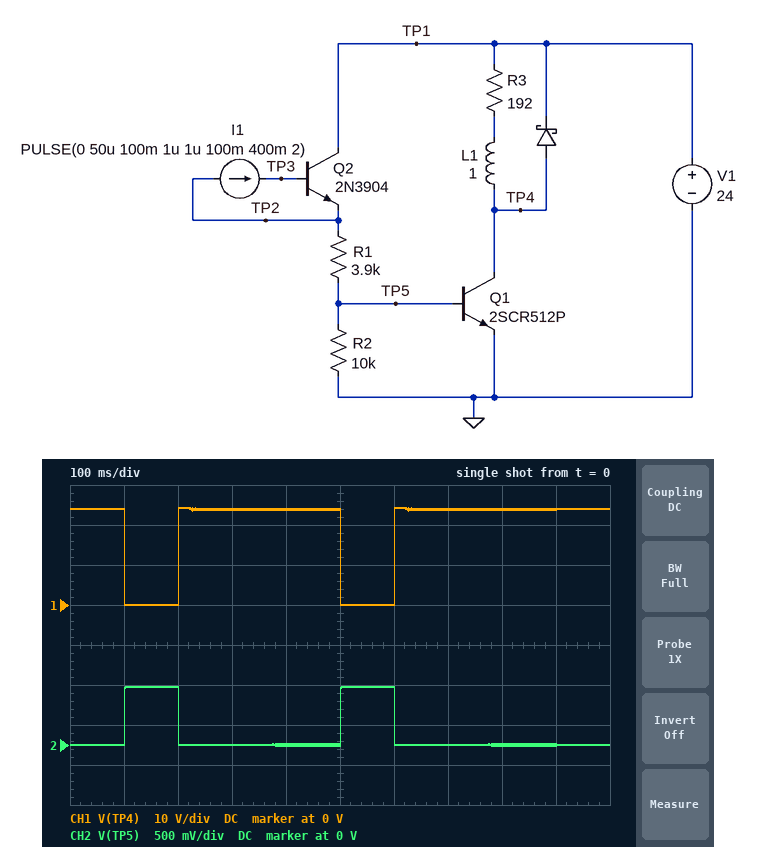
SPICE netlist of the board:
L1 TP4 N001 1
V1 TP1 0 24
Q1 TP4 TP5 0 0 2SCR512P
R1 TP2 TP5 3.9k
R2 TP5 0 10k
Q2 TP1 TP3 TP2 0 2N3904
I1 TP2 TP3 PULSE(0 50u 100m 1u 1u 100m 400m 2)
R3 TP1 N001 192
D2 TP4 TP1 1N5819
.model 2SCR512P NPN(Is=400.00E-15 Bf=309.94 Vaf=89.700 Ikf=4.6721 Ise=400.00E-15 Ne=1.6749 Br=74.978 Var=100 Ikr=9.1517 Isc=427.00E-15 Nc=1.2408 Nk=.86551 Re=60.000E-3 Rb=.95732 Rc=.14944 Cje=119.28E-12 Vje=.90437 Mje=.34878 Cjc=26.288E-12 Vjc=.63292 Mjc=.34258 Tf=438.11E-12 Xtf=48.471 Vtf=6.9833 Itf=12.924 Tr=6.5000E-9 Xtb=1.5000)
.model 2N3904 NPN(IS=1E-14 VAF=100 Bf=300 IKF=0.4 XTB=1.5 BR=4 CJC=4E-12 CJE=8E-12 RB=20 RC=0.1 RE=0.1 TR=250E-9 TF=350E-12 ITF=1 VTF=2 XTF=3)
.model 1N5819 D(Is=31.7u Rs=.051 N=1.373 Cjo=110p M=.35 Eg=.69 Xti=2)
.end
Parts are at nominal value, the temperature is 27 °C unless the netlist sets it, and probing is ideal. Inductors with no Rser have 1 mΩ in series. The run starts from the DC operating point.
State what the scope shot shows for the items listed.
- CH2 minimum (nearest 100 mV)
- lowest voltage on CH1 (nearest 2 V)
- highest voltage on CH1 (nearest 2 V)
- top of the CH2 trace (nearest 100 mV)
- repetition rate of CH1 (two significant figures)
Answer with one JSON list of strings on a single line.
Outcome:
["0 V", "0 V", "24 V", "700 mV", "2.5 Hz"]
